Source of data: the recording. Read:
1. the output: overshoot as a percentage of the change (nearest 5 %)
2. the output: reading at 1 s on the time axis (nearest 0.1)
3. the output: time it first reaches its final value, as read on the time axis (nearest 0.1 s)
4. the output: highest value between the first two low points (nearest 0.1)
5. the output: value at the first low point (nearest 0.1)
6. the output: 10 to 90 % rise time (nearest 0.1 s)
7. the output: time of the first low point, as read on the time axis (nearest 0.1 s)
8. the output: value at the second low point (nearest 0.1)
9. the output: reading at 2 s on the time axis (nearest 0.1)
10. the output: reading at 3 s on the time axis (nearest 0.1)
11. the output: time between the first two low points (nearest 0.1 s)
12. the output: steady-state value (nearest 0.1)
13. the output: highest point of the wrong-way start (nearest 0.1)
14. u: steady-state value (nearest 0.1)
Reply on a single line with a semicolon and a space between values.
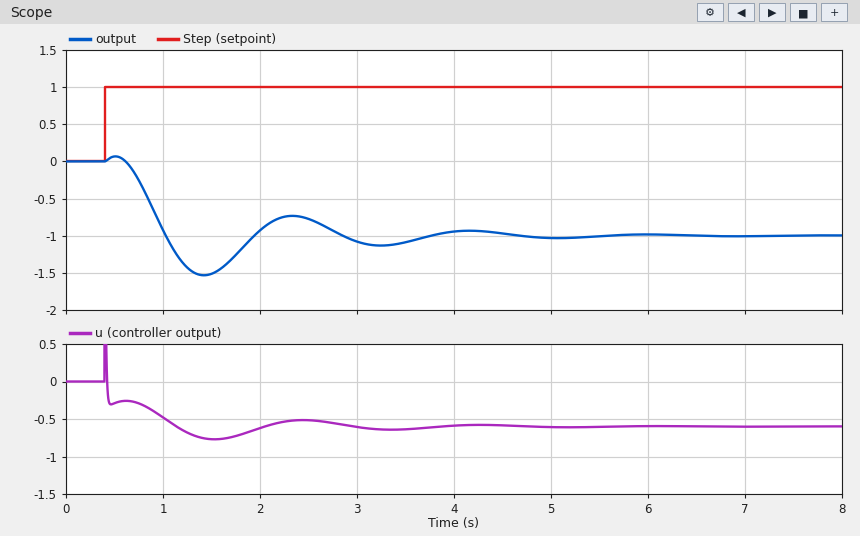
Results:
55 %; -0.9; 1.0 s; -0.7; -1.5; 0.3 s; 1.4 s; -1.1; -0.9; -1.1; 1.8 s; -1.0; 0.1; -0.6
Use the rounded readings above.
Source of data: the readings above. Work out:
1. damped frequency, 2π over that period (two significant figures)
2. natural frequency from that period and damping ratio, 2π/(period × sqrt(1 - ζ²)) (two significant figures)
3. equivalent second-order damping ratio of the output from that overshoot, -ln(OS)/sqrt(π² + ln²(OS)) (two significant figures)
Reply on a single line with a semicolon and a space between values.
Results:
3.5 rad/s; 3.6 rad/s; 0.19
